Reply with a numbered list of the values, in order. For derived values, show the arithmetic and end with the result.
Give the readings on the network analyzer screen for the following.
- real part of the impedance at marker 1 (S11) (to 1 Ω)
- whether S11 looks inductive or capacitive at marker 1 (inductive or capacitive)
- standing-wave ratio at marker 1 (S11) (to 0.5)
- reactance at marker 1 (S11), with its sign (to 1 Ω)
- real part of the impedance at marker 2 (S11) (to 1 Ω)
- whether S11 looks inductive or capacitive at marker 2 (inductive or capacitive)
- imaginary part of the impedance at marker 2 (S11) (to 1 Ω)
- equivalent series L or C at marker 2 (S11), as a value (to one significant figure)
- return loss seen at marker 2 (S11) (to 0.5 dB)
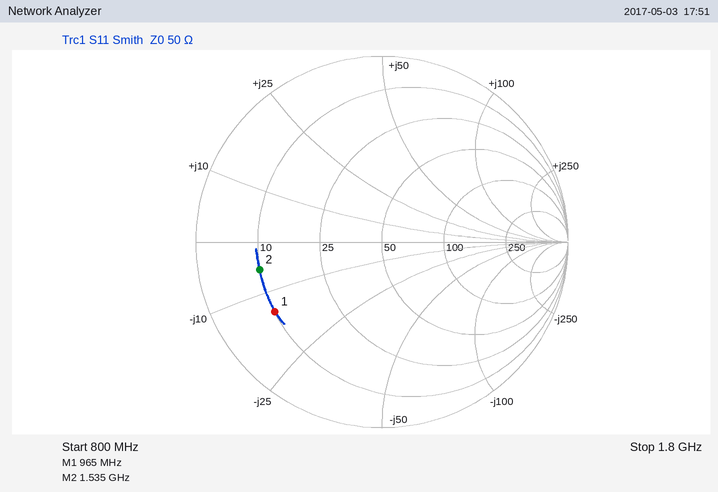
1. 10 Ω
2. capacitive
3. 5.5
4. -14 Ω
5. 10 Ω
6. capacitive
7. -5 Ω
8. C = 1/(2π × 1.535 GHz × 5 Ω) ≈ 20.7 pF, so 20 pF to one significant figure
9. 3.5 dB
